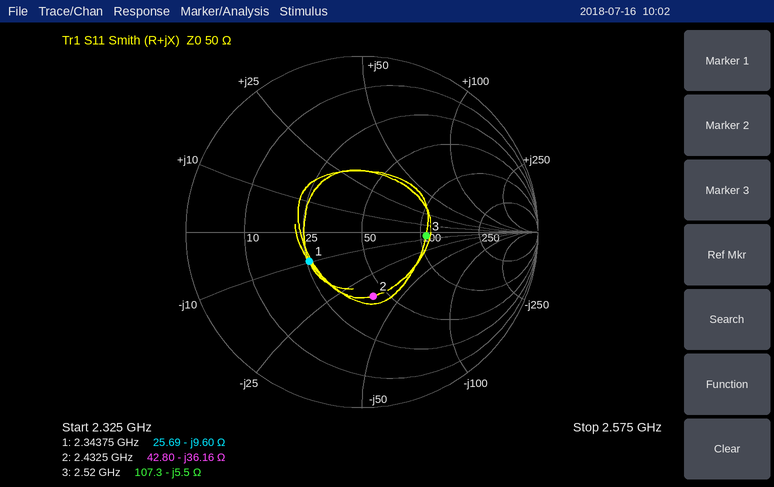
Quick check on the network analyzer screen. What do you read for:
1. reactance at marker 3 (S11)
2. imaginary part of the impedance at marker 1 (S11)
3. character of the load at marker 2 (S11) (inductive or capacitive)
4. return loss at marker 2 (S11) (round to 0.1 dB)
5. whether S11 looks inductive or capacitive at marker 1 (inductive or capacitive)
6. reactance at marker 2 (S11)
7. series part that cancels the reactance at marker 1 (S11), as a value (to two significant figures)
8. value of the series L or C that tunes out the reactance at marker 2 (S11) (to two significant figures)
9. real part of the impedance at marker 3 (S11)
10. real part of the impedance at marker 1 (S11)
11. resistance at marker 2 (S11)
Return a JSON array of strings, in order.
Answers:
["-5.5 Ω", "-9.60 Ω", "capacitive", "8.6 dB", "capacitive", "-36.16 Ω", "650 pH", "2.4 nH", "107.3 Ω", "25.69 Ω", "42.80 Ω"]
